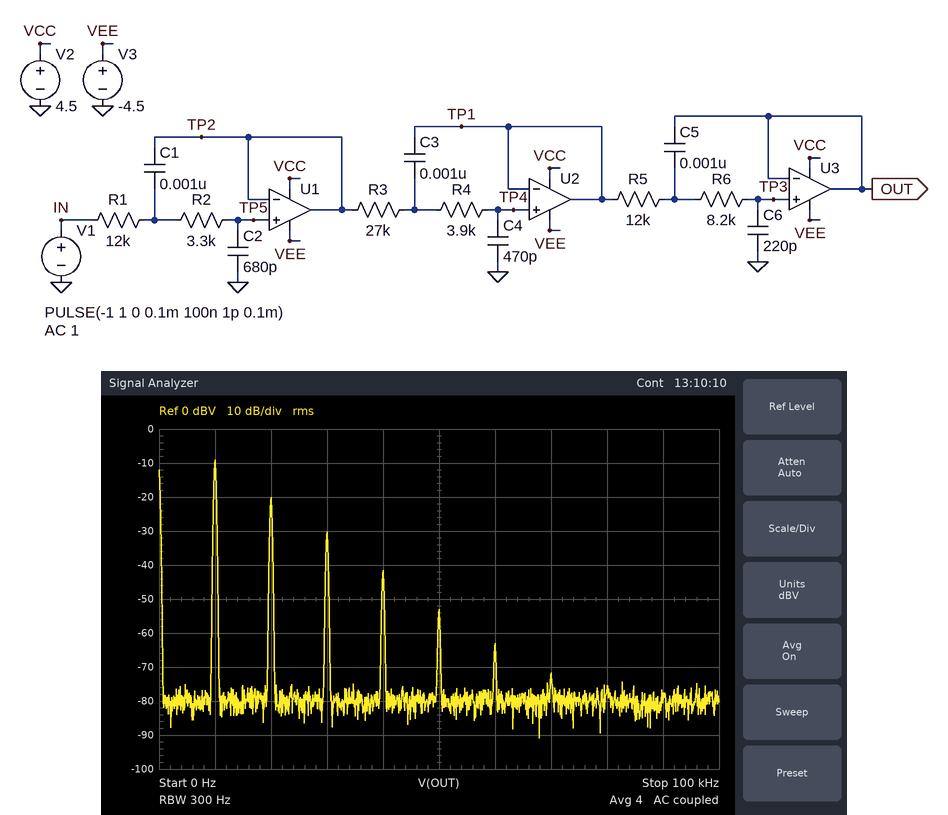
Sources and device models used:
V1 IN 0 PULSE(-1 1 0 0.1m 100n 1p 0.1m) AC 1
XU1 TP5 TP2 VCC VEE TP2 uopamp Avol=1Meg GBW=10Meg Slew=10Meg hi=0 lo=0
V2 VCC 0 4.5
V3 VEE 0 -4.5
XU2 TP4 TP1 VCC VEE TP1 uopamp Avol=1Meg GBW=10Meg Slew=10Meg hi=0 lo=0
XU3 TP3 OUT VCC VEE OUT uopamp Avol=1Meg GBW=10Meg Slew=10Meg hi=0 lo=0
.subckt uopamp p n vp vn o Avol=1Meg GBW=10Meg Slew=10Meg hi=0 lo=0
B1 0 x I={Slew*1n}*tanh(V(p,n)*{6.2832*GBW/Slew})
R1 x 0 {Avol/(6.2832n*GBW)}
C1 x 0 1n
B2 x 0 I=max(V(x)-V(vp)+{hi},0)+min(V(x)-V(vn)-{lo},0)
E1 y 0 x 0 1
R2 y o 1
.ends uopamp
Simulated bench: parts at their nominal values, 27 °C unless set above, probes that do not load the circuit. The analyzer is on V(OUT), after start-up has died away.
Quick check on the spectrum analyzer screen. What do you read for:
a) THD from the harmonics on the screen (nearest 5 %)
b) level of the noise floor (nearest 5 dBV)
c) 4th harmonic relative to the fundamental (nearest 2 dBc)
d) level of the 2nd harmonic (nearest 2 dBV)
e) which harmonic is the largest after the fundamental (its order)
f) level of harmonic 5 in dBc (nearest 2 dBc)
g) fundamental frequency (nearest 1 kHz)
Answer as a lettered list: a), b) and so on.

a) 30 %
b) -80 dBV
c) -32 dBc
d) -20 dBV
e) 2
f) -44 dBc
g) 10 kHz
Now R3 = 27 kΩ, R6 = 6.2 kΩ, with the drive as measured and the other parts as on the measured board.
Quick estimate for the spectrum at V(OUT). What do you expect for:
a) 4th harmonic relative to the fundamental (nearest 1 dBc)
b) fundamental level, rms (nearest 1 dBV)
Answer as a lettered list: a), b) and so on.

a) -31 dBc
b) -9 dBV
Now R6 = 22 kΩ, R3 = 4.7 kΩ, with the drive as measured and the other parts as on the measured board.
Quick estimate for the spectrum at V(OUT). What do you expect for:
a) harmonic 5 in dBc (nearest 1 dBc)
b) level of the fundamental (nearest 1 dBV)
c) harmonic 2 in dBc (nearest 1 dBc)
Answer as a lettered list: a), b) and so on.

a) -42 dBc
b) -7 dBV
c) -9 dBc
